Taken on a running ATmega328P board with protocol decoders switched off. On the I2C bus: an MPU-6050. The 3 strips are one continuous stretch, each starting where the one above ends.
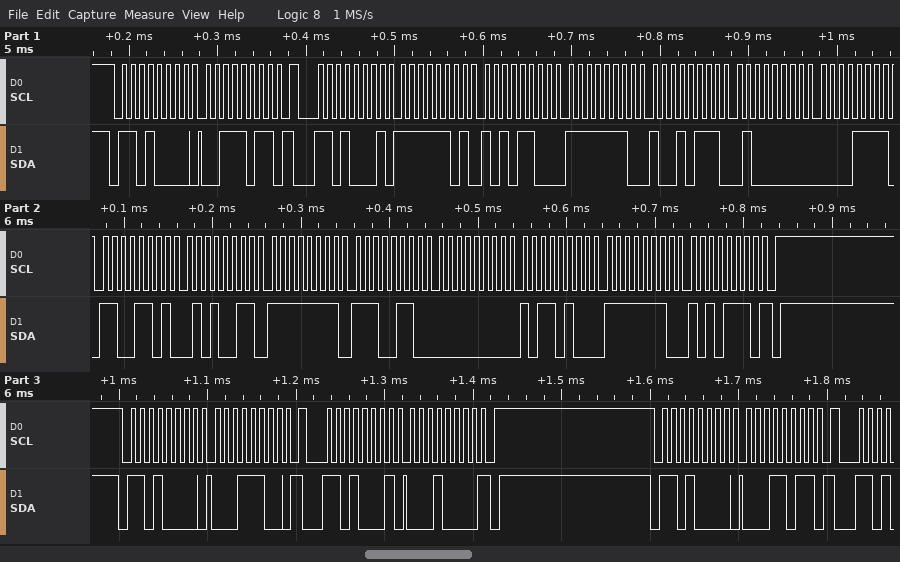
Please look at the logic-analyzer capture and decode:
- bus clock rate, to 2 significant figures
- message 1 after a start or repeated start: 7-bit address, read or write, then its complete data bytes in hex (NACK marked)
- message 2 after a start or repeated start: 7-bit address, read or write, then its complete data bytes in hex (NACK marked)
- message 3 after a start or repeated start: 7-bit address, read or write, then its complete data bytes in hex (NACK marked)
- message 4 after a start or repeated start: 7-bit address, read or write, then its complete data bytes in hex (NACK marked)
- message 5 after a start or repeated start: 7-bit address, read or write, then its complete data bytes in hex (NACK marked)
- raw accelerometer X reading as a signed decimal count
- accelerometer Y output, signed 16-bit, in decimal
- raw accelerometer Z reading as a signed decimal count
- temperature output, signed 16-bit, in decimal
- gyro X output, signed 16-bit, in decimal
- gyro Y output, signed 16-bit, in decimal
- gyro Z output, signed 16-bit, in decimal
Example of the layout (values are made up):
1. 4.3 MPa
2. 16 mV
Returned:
1. 100 kHz
2. 0x68 write: 3B
3. 0x68 read: FD AC FE 97 40 0F CD 53 FF E6 00 B4 FE AE NACK
4. 0x68 write: 1C
5. 0x68 read: 10 NACK
6. 0x68 write: 1B
7. -596
8. -361
9. 16399
10. -12973
11. -26
12. 180
13. -338
